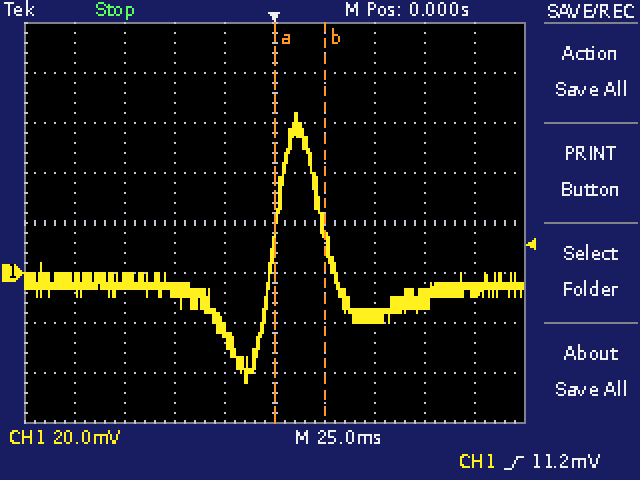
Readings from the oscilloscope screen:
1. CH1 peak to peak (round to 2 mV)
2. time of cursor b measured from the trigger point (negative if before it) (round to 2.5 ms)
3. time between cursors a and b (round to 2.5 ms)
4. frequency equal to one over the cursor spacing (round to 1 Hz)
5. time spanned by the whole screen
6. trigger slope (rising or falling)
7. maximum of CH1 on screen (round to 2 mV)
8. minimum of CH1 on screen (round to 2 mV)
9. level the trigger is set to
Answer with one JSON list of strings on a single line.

["108 mV", "+25.0 ms", "25.0 ms", "40 Hz", "250 ms", "rising", "64 mV", "-44 mV", "11.2 mV"]
